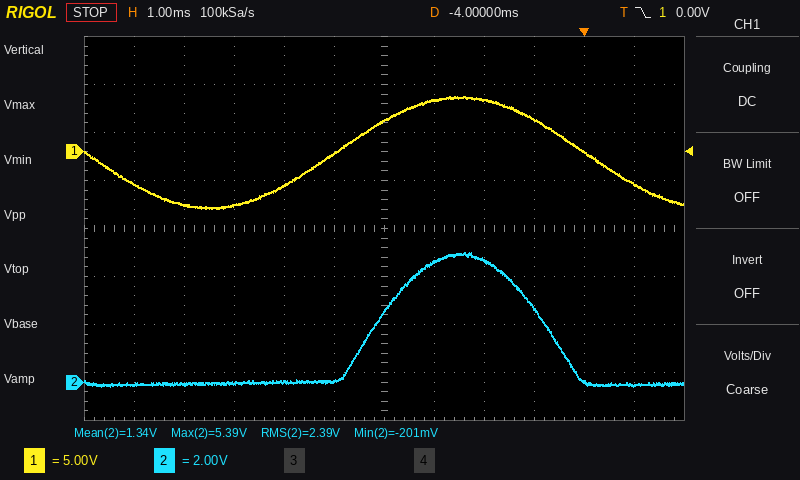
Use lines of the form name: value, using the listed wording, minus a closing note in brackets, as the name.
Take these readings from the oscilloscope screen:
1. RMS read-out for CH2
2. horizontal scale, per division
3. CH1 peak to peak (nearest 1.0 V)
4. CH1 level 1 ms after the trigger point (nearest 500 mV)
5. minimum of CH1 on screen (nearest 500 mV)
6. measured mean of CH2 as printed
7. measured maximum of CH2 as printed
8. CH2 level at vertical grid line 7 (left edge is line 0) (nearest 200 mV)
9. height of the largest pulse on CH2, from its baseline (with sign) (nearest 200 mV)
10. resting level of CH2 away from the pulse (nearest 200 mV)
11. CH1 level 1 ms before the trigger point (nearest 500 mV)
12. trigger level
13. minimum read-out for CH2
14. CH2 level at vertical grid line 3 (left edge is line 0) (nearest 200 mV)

RMS read-out for CH2: 2.39 V
horizontal scale, per division: 1 ms
CH1 peak to peak: 12.0 V
CH1 level 1 ms after the trigger point: -3.5 V
minimum of CH1 on screen: -6.0 V
measured mean of CH2 as printed: 1.34 V
measured maximum of CH2 as printed: 5.39 V
CH2 level at vertical grid line 7 (left edge is line 0): 5.0 V
height of the largest pulse on CH2, from its baseline (with sign): +5.4 V
resting level of CH2 away from the pulse: 0.0 V
CH1 level 1 ms before the trigger point: 3.5 V
trigger level: 0.00 V
minimum read-out for CH2: -201 mV
CH2 level at vertical grid line 3 (left edge is line 0): 0.0 V
